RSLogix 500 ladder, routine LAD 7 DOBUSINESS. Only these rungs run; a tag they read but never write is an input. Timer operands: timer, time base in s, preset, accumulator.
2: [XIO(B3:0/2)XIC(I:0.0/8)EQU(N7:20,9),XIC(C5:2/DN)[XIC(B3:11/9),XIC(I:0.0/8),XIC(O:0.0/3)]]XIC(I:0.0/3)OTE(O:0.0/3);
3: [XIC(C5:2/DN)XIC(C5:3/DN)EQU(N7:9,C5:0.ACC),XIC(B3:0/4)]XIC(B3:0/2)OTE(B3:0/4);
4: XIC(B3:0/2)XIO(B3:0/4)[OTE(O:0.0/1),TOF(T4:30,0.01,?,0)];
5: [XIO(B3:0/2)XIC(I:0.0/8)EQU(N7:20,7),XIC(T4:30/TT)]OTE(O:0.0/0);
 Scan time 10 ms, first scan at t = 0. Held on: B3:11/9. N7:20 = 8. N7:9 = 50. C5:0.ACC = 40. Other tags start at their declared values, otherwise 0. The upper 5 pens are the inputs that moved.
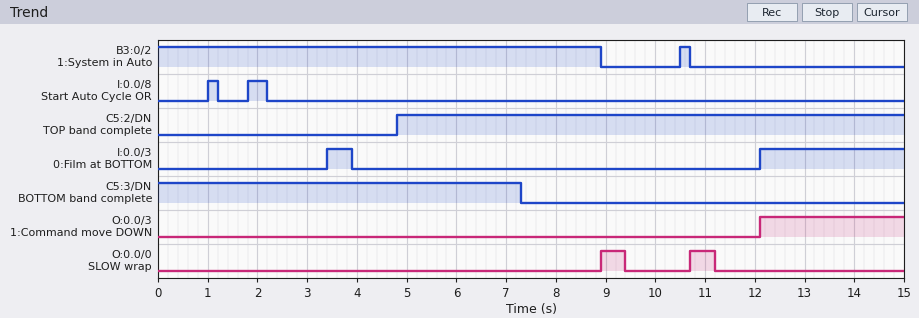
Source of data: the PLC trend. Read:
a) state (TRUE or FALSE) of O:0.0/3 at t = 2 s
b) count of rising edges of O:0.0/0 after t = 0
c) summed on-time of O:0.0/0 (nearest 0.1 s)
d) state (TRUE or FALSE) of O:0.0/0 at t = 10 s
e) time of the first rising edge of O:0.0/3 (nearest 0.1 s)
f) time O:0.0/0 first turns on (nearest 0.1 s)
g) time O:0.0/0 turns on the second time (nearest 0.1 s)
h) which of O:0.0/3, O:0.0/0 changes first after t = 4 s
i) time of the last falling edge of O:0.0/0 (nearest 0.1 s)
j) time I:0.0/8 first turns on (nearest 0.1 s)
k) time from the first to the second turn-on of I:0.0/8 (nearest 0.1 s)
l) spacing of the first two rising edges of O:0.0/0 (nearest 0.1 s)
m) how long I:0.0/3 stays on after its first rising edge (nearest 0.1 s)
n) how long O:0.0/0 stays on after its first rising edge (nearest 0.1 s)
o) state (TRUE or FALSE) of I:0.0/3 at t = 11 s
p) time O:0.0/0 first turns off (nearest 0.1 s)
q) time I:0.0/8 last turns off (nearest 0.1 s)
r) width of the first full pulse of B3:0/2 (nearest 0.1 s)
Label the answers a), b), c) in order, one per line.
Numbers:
a) FALSE
b) 2
c) 1.0 s
d) FALSE
e) 12.1 s
f) 8.9 s
g) 10.7 s
h) O:0.0/0
i) 11.2 s
j) 1.0 s
k) 0.8 s
l) 1.8 s
m) 0.5 s
n) 0.5 s
o) FALSE
p) 9.4 s
q) 2.2 s
r) 0.2 s
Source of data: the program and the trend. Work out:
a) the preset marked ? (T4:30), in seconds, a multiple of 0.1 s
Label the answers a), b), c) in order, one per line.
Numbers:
a) 0.5 s
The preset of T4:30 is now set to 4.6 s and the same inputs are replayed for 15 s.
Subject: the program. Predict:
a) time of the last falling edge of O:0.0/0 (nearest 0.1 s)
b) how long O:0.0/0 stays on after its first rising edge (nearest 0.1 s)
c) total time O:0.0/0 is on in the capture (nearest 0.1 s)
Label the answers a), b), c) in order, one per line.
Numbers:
a) 10.5 s
b) 1.6 s
c) 5.9 s
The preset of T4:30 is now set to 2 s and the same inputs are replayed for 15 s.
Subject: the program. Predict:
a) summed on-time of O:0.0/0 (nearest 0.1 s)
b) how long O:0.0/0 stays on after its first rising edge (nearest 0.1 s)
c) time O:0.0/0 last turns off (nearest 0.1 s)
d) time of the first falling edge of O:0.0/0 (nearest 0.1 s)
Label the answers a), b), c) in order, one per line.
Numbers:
a) 3.6 s
b) 1.6 s
c) 12.7 s
d) 10.5 s
